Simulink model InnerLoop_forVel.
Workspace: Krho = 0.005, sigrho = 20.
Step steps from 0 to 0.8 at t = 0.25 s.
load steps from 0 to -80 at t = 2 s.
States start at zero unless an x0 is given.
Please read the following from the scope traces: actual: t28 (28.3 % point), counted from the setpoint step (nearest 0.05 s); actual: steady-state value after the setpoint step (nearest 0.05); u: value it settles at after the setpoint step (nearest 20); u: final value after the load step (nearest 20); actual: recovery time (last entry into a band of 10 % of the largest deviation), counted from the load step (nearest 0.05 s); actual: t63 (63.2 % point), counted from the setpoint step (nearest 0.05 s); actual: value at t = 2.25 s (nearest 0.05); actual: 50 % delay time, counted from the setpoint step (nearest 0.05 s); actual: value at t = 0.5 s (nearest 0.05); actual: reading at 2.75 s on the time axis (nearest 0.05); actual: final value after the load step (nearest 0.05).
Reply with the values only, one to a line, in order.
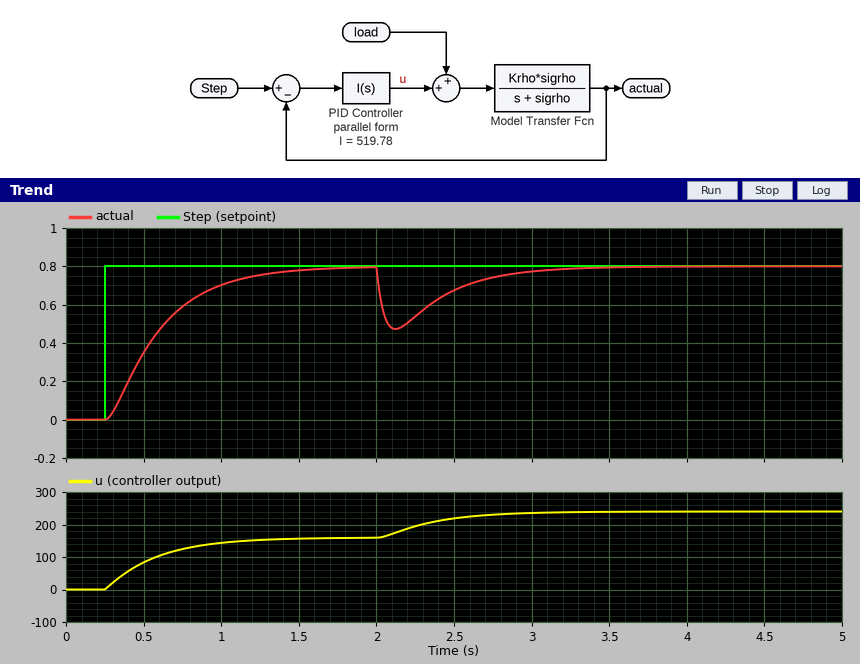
0.15 s
0.80
160
240
0.95 s
0.40 s
0.55
0.30 s
0.35
0.75
0.80
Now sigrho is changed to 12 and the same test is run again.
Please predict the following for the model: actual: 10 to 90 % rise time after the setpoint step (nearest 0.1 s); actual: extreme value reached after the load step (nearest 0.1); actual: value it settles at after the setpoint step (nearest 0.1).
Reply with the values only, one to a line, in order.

0.7 s
0.5
0.8
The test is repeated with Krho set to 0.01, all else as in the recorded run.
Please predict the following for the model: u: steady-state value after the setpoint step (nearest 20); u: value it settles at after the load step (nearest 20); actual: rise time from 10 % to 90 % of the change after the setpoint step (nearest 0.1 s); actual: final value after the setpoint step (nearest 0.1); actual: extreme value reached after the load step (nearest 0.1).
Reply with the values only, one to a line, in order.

80
160
0.3 s
0.8
0.2
